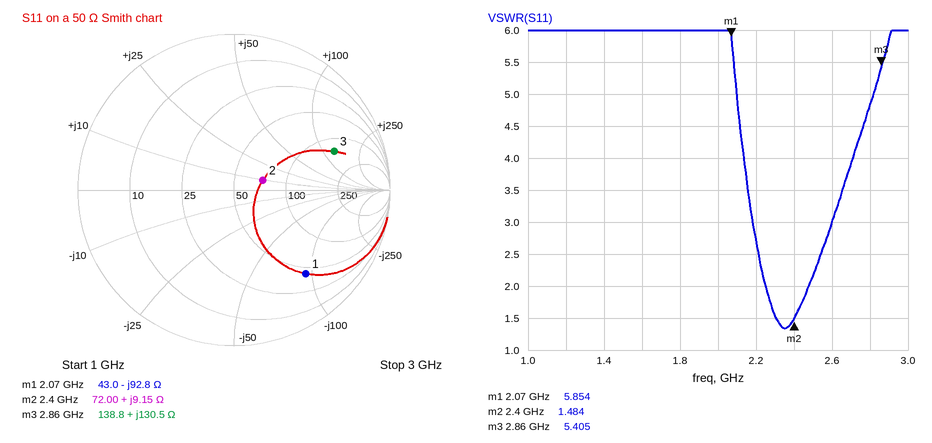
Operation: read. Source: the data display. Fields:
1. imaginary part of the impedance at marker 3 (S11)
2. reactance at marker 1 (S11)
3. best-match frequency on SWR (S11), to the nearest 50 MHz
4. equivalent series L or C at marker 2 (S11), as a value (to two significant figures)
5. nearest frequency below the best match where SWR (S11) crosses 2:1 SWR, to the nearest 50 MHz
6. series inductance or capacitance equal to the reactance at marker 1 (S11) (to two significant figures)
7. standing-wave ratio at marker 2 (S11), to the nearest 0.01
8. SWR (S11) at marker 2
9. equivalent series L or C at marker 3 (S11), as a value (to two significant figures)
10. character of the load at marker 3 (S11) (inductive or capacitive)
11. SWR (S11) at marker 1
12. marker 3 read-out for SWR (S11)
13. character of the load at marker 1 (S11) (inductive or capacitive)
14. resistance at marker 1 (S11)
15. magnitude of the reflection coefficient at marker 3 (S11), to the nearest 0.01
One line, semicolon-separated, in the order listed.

+130.5 Ω; -92.8 Ω; 2.35 GHz; 610 pH; 2.25 GHz; 830 fF; 1.48; 1.484; 7.3 nH; inductive; 5.854; 5.405; capacitive; 43.0 Ω; 0.69
